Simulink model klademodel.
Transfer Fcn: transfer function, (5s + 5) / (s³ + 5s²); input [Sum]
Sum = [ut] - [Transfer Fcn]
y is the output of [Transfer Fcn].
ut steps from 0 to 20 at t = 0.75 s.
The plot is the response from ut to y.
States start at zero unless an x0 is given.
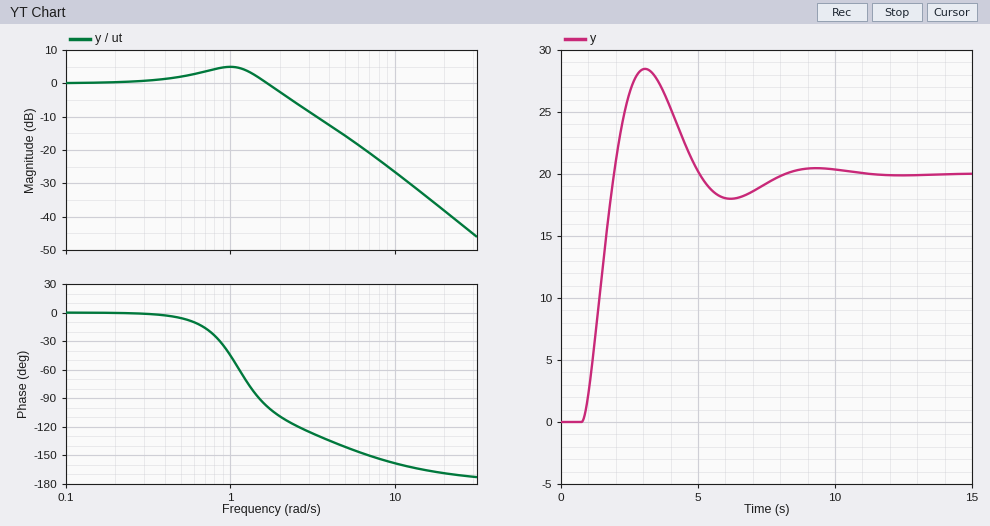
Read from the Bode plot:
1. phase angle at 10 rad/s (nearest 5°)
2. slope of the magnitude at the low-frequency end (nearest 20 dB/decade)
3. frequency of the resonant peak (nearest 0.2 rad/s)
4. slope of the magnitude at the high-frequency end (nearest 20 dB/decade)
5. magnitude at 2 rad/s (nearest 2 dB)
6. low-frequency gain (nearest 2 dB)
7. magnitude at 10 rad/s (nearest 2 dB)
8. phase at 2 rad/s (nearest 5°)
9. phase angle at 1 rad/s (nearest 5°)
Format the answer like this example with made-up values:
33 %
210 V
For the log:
-160°
0 dB/decade
1.0 rad/s
-40 dB/decade
-2 dB
0 dB
-26 dB
-110°
-45°
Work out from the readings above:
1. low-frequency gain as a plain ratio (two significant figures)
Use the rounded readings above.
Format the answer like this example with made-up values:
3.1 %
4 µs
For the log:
1.0
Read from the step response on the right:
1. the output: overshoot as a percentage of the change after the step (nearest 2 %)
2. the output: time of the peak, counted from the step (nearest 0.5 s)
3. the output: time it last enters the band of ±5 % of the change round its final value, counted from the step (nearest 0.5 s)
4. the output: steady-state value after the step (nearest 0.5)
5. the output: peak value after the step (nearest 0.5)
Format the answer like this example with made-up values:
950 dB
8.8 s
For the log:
42 %
2.5 s
6.5 s
20.0
28.5
